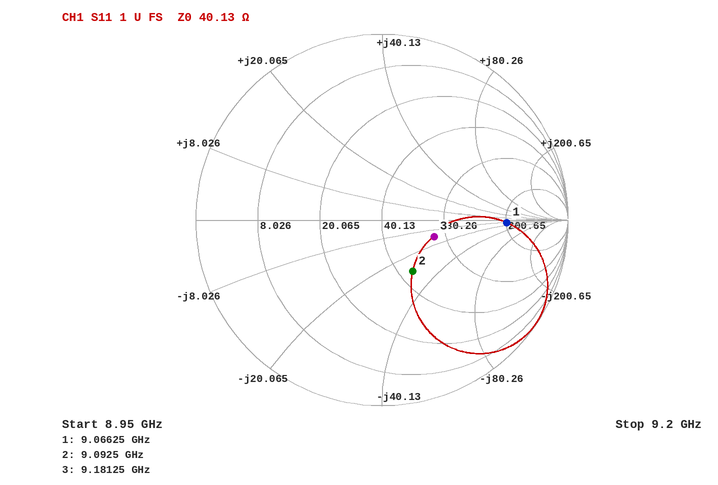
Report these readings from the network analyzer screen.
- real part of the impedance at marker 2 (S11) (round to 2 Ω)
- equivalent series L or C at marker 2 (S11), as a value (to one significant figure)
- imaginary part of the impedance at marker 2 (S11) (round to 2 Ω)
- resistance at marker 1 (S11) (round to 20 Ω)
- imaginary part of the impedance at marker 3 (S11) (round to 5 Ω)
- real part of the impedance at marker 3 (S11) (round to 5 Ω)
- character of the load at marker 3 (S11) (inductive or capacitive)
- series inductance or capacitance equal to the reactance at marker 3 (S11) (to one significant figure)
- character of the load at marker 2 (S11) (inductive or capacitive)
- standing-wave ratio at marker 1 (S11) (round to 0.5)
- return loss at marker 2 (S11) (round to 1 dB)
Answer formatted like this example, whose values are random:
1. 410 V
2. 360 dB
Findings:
1. 46 Ω
2. 600 fF
3. -28 Ω
4. 200 Ω
5. -15 Ω
6. 70 Ω
7. capacitive
8. 1 pF
9. capacitive
10. 5.0
11. 10 dB
